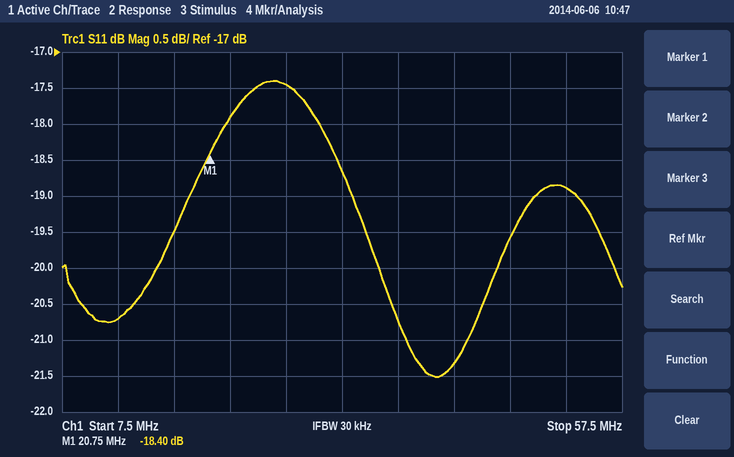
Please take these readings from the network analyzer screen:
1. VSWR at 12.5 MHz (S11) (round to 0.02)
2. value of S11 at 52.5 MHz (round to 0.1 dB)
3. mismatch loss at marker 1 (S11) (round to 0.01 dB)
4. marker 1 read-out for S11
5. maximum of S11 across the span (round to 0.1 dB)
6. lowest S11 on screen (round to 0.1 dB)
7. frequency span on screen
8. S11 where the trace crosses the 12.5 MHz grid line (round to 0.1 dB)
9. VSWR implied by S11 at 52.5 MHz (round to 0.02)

1.20
-18.9 dB
0.06 dB
-18.40 dB
-17.4 dB
-21.5 dB
50 MHz
-20.7 dB
1.26
